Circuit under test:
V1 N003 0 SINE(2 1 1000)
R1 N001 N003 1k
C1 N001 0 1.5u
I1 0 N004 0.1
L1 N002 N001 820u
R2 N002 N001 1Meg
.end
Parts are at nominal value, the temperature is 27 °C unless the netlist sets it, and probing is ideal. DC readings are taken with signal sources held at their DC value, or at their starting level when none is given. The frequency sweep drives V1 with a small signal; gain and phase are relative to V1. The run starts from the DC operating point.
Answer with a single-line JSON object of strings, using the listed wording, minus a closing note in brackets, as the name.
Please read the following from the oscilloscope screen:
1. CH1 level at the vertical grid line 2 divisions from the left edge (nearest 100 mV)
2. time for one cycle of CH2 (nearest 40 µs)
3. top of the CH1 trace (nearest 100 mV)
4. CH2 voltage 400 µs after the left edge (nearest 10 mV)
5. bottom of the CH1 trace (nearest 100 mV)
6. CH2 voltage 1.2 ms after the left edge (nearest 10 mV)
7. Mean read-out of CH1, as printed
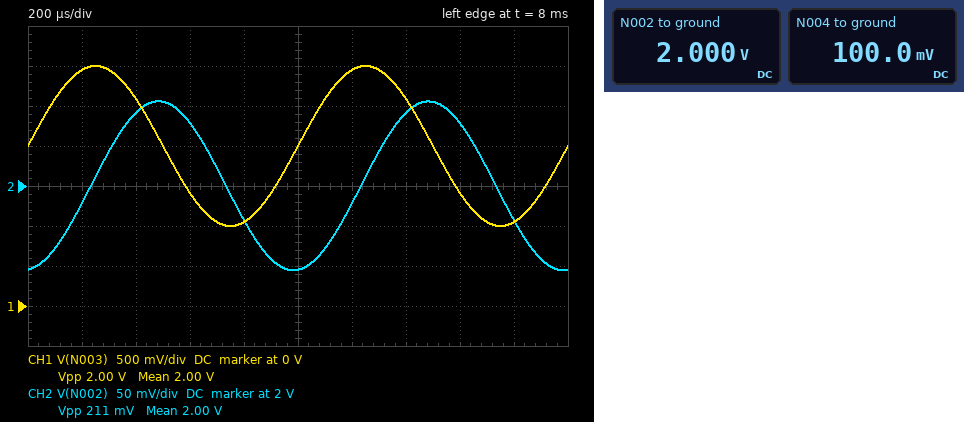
{"CH1 level at the vertical grid line 2 divisions from the left edge": "2.6 V", "time for one cycle of CH2": "1.00 ms", "top of the CH1 trace": "3.0 V", "CH2 voltage 400 µs after the left edge": "2.09 V", "bottom of the CH1 trace": "1.0 V", "CH2 voltage 1.2 ms after the left edge": "1.98 V", "Mean read-out of CH1, as printed": "2.00 V"}
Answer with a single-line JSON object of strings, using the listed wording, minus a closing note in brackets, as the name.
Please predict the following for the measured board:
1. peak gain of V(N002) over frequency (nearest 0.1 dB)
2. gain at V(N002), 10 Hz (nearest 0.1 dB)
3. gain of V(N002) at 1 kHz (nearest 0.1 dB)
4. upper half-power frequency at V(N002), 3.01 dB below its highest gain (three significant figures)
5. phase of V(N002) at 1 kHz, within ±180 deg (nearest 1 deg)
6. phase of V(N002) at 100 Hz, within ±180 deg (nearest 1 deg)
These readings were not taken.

{"peak gain of V(N002) over frequency": "0 dB", "gain at V(N002), 10 Hz": "0 dB", "gain of V(N002) at 1 kHz": "-19.5 dB", "upper half-power frequency at V(N002), 3.01 dB below its highest gain": "106 Hz", "phase of V(N002) at 1 kHz, within ±180 deg": "-84 deg", "phase of V(N002) at 100 Hz, within ±180 deg": "-43 deg"}
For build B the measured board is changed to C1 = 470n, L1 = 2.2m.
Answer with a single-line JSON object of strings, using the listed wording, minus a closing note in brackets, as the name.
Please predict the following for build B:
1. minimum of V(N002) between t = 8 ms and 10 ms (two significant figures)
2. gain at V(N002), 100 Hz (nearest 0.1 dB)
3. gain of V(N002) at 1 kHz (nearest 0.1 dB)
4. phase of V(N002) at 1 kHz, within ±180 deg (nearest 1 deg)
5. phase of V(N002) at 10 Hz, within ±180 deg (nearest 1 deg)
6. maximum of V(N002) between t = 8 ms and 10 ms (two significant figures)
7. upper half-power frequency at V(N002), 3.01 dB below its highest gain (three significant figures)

{"minimum of V(N002) between t = 8 ms and 10 ms": "1.7 V", "gain at V(N002), 100 Hz": "-0.4 dB", "gain of V(N002) at 1 kHz": "-9.9 dB", "phase of V(N002) at 1 kHz, within ±180 deg": "-71 deg", "phase of V(N002) at 10 Hz, within ±180 deg": "-2 deg", "maximum of V(N002) between t = 8 ms and 10 ms": "2.3 V", "upper half-power frequency at V(N002), 3.01 dB below its highest gain": "339 Hz"}
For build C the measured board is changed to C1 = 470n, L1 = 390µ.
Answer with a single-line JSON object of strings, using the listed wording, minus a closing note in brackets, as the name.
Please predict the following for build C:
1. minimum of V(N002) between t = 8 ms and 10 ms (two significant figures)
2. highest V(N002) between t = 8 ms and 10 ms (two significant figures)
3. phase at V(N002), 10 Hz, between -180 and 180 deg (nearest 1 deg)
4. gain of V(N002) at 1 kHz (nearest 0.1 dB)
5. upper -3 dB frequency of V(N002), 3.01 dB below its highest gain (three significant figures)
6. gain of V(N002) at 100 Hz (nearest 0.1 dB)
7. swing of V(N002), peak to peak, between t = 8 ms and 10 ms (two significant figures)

{"minimum of V(N002) between t = 8 ms and 10 ms": "1.7 V", "highest V(N002) between t = 8 ms and 10 ms": "2.3 V", "phase at V(N002), 10 Hz, between -180 and 180 deg": "-2 deg", "gain of V(N002) at 1 kHz": "-9.9 dB", "upper -3 dB frequency of V(N002), 3.01 dB below its highest gain": "339 Hz", "gain of V(N002) at 100 Hz": "-0.4 dB", "swing of V(N002), peak to peak, between t = 8 ms and 10 ms": "640 mV"}
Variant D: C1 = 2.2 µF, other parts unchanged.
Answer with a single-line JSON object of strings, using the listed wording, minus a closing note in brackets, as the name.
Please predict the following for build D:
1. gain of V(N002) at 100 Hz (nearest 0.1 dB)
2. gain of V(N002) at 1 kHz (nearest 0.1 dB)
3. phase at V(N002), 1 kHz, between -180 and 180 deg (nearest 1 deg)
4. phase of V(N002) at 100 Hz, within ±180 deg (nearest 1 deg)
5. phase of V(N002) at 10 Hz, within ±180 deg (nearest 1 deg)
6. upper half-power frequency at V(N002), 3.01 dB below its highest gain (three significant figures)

{"gain of V(N002) at 100 Hz": "-4.6 dB", "gain of V(N002) at 1 kHz": "-22.8 dB", "phase at V(N002), 1 kHz, between -180 and 180 deg": "-86 deg", "phase of V(N002) at 100 Hz, within ±180 deg": "-54 deg", "phase of V(N002) at 10 Hz, within ±180 deg": "-8 deg", "upper half-power frequency at V(N002), 3.01 dB below its highest gain": "72.3 Hz"}
